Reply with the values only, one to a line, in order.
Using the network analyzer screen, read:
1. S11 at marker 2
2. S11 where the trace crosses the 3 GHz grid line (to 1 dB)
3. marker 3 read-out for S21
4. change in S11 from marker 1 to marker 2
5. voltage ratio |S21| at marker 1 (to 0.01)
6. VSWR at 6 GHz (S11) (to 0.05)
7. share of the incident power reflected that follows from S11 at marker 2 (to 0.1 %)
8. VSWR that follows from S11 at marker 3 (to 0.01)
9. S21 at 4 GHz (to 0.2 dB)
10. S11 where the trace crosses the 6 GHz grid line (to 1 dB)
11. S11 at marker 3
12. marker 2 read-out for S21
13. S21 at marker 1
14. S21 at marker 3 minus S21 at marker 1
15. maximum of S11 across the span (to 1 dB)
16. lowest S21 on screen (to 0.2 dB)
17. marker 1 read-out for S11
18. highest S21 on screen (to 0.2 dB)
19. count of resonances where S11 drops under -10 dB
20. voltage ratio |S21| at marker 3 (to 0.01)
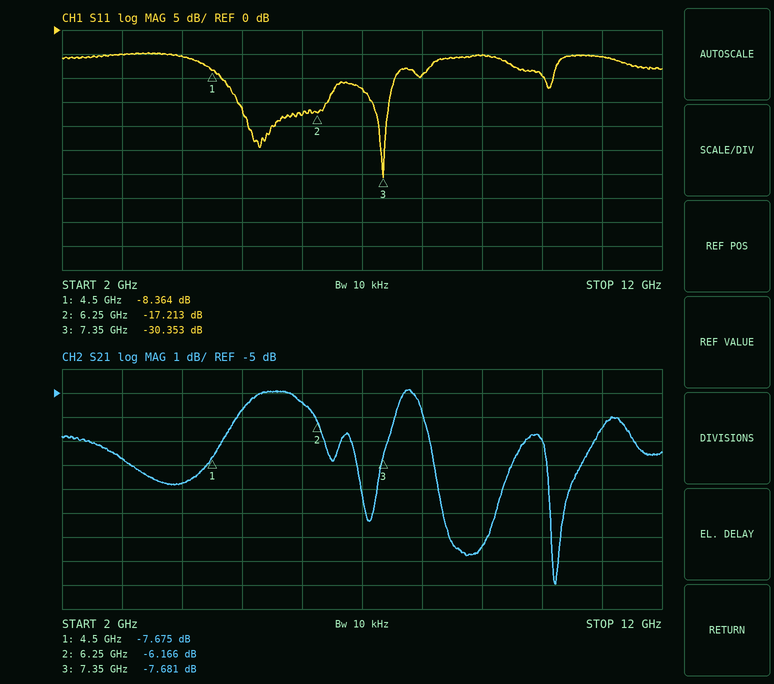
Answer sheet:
-17.213 dB
-5 dB
-7.681 dB
-8.849 dB
0.41
1.30
1.9 %
1.06
-8.8 dB
-18 dB
-30.353 dB
-6.166 dB
-7.675 dB
-0.006 dB
-5 dB
-13.0 dB
-8.364 dB
-4.8 dB
3
0.41
